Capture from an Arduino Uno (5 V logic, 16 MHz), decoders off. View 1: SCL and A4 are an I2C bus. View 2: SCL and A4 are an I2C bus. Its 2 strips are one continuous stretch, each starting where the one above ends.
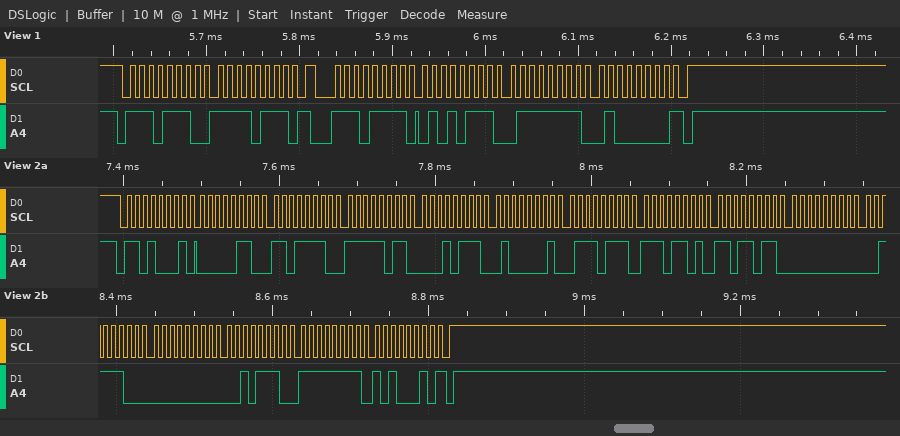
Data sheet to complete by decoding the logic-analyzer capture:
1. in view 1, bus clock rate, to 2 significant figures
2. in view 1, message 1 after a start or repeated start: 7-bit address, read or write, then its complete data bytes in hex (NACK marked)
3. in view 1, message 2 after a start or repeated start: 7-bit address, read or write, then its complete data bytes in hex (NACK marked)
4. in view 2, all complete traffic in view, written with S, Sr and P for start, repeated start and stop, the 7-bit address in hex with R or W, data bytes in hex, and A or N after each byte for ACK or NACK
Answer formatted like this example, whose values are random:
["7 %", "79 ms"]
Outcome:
["100 kHz", "0x77 write: F7", "0x77 read: 57 7F 40 NACK", "S 68R A 06 A DE A FB A 17 A 41 A 77 A ED A DB A 00 A 3C A 00 A 2E A FF A A2 N P"]
